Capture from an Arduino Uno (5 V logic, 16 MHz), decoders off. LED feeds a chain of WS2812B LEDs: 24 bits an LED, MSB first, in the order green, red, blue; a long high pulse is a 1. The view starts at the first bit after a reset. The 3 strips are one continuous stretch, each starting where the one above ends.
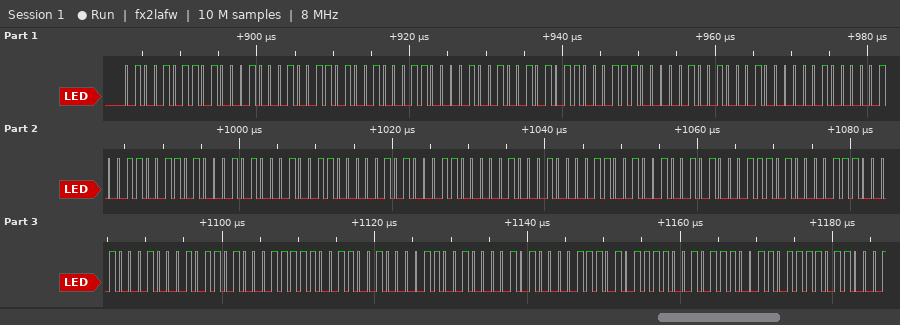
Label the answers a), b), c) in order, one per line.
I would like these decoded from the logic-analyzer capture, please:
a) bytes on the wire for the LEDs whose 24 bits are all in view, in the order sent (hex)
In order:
a) 4B 44 4D 23 09 2B 1C 12 20 41 33 45 13 05 18 22 19 25 1D 0E 22 2D 1F 32 19 0A 1D 79 73 7B
